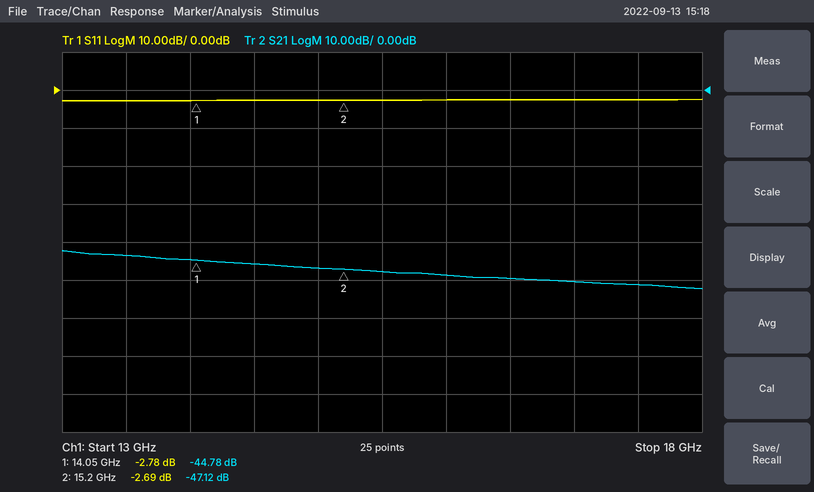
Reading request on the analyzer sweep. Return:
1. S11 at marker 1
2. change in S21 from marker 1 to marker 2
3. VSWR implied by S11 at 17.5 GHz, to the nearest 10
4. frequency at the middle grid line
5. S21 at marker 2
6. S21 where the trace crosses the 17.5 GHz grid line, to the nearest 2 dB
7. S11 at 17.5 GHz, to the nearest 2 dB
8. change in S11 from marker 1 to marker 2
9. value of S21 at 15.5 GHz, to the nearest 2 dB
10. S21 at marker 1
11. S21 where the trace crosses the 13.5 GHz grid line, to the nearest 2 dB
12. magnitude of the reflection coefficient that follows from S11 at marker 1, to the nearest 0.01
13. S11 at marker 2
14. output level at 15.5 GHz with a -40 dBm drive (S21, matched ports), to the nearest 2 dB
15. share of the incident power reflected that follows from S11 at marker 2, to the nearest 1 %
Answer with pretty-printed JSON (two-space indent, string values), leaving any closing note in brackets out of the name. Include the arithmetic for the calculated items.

{
  "S11 at marker 1": "-2.78 dB",
  "change in S21 from marker 1 to marker 2": "-47.12 − (-44.78) = -2.34 dB",
  "VSWR implied by S11 at 17.5 GHz, to the nearest 10": "|Γ| = 10^(-2/20) = 0.7943; VSWR = (1 + 0.7943)/(1 − 0.7943) ≈ 8.72, so 10 to the nearest 10",
  "frequency at the middle grid line": "15.5 GHz",
  "S21 at marker 2": "-47.12 dB",
  "S21 where the trace crosses the 17.5 GHz grid line, to the nearest 2 dB": "-52 dB",
  "S11 at 17.5 GHz, to the nearest 2 dB": "-2 dB",
  "change in S11 from marker 1 to marker 2": "-2.69 − (-2.78) = 0.09 dB",
  "value of S21 at 15.5 GHz, to the nearest 2 dB": "-48 dB",
  "S21 at marker 1": "-44.78 dB",
  "S21 where the trace crosses the 13.5 GHz grid line, to the nearest 2 dB": "-44 dB",
  "magnitude of the reflection coefficient that follows from S11 at marker 1, to the nearest 0.01": "10^(-2.78/20) ≈ 0.73",
  "S11 at marker 2": "-2.69 dB",
  "output level at 15.5 GHz with a -40 dBm drive (S21, matched ports), to the nearest 2 dB": "-40 dBm + (-48 dB) = -88 dBm",
  "share of the incident power reflected that follows from S11 at marker 2, to the nearest 1 %": "10^(-2.69/10) ≈ 54 %"
}
